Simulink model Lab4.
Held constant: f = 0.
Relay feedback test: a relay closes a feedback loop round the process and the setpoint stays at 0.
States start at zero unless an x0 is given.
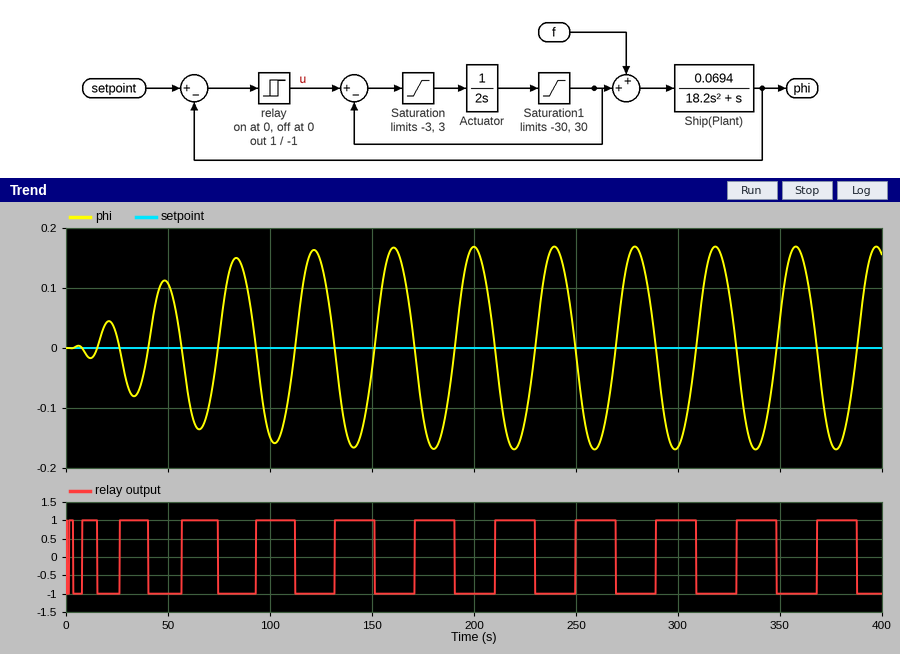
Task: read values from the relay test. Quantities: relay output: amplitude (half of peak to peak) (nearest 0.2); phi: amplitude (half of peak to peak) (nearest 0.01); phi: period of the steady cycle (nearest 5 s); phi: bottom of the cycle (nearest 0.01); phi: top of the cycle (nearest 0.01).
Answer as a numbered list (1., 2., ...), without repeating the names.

1. 1.0
2. 0.17
3. 40 s
4. -0.17
5. 0.17
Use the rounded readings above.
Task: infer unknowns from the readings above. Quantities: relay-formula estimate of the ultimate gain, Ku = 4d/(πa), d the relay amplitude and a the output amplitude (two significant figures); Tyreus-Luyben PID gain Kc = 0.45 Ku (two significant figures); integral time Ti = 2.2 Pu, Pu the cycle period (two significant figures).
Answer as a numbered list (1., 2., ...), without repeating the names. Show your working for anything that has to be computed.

1. 4 × 1 / (π × 0.17) = 7.5
2. 0.45 × 7.5 = 3.4
3. 2.2 × 40 = 88 s
